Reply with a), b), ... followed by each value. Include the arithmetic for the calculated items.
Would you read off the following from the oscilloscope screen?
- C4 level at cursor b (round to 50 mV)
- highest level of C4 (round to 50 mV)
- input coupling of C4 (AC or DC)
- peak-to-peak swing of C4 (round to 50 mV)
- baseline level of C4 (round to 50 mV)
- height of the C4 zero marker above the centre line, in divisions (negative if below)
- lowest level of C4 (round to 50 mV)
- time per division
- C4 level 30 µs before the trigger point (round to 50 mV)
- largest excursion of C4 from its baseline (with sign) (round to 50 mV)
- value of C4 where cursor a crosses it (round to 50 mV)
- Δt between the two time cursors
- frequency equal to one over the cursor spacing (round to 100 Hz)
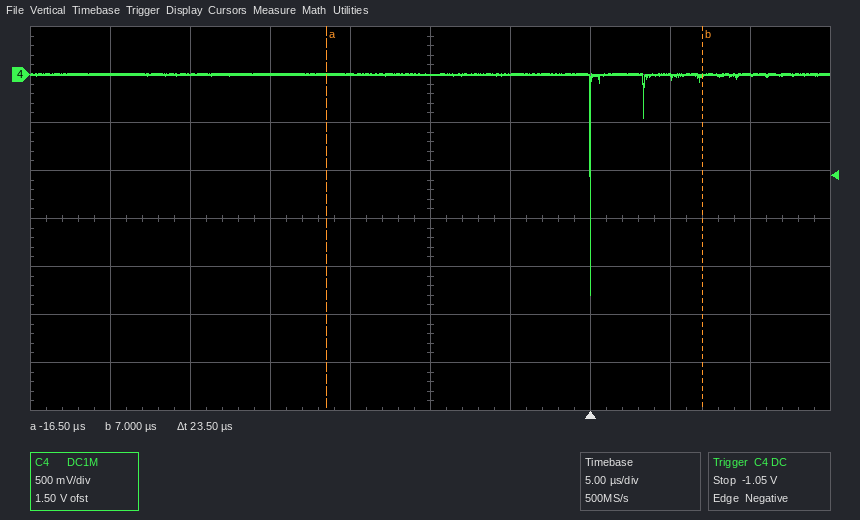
a) -50 mV
b) 0 mV
c) DC
d) 0 mV − (-2.30 V) = 2.30 V
e) 0 mV
f) +3.0 div
g) -2.30 V
h) 5 µs
i) 0 mV
j) -2.30 V − (0 mV) = -2.30 V
k) 0 mV
l) 23.5 µs
m) 1 / 23.5 µs ≈ 42.6 kHz
